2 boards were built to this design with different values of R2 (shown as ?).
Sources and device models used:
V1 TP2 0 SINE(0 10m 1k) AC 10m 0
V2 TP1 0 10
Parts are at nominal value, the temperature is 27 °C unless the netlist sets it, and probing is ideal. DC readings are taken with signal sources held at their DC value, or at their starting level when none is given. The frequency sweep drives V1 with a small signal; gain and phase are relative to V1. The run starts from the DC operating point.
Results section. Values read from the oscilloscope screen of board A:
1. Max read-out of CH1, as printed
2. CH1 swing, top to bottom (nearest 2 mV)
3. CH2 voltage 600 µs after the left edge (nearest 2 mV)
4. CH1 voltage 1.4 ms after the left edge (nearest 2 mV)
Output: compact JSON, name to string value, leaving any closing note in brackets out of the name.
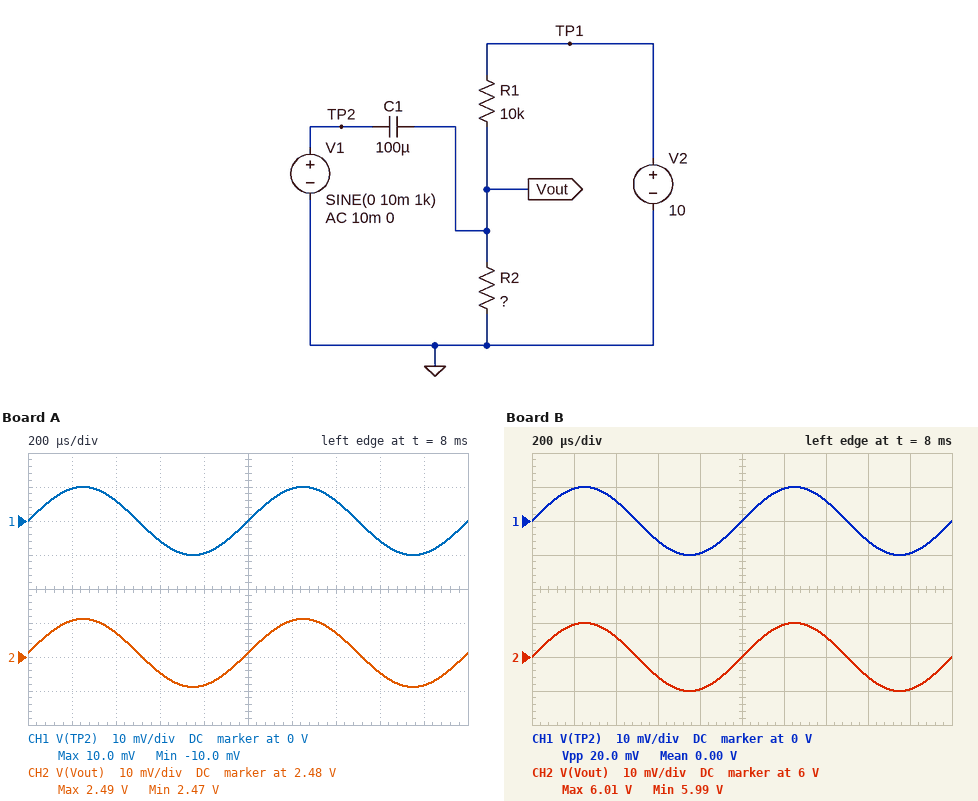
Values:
{"Max read-out of CH1, as printed": "10.0 mV", "CH1 swing, top to bottom": "20 mV", "CH2 voltage 600 µs after the left edge": "2.476 V", "CH1 voltage 1.4 ms after the left edge": "6 mV"}
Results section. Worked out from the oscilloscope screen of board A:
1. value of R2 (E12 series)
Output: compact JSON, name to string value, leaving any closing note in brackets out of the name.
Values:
{"value of R2": "3.3 kΩ"}
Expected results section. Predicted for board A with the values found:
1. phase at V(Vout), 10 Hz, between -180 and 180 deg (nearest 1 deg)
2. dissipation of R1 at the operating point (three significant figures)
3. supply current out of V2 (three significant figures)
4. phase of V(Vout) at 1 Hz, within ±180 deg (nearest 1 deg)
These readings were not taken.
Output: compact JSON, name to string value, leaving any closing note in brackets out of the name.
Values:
{"phase at V(Vout), 10 Hz, between -180 and 180 deg": "4 deg", "dissipation of R1 at the operating point": "5.65 mW", "supply current out of V2": "752 µA", "phase of V(Vout) at 1 Hz, within ±180 deg": "33 deg"}
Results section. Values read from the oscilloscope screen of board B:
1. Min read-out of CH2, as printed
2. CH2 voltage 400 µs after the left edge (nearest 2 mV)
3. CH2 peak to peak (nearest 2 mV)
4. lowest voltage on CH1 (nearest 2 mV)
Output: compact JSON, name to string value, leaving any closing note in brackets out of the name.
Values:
{"Min read-out of CH2, as printed": "5.99 V", "CH2 voltage 400 µs after the left edge": "6.006 V", "CH2 peak to peak": "20 mV", "lowest voltage on CH1": "-10 mV"}
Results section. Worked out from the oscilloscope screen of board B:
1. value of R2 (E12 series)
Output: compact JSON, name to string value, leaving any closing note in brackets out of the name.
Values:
{"value of R2": "15 kΩ"}
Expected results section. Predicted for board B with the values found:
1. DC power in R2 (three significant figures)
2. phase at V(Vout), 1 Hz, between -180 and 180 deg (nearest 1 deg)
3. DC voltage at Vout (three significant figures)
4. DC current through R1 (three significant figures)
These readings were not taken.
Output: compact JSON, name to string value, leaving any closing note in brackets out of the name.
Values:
{"DC power in R2": "2.40 mW", "phase at V(Vout), 1 Hz, between -180 and 180 deg": "15 deg", "DC voltage at Vout": "6.00 V", "DC current through R1": "400 µA"}
